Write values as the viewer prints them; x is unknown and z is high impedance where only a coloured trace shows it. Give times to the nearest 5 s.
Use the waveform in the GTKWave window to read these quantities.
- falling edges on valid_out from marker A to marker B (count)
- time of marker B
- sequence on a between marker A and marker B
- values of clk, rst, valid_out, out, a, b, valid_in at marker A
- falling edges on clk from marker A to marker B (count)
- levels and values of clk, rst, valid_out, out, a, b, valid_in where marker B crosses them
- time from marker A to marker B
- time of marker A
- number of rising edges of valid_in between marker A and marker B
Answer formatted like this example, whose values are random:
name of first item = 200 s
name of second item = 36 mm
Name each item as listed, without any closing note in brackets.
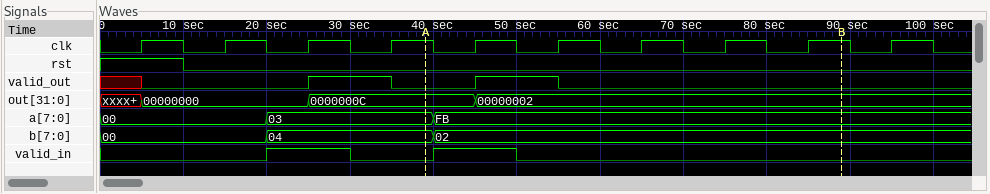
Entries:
falling edges on valid_out from marker A to marker B = 1
time of marker B = 90 s
sequence on a between marker A and marker B = 03, FB
values of clk, rst, valid_out, out, a, b, valid_in at marker A = clk=1, rst=0, valid_out=0, out=0000000C, a=03, b=04, valid_in=0
falling edges on clk from marker A to marker B = 5
levels and values of clk, rst, valid_out, out, a, b, valid_in where marker B crosses them = clk=1, rst=0, valid_out=0, out=00000002, a=FB, b=02, valid_in=0
time from marker A to marker B = 50 s
time of marker A = 40 s
number of rising edges of valid_in between marker A and marker B = 1
